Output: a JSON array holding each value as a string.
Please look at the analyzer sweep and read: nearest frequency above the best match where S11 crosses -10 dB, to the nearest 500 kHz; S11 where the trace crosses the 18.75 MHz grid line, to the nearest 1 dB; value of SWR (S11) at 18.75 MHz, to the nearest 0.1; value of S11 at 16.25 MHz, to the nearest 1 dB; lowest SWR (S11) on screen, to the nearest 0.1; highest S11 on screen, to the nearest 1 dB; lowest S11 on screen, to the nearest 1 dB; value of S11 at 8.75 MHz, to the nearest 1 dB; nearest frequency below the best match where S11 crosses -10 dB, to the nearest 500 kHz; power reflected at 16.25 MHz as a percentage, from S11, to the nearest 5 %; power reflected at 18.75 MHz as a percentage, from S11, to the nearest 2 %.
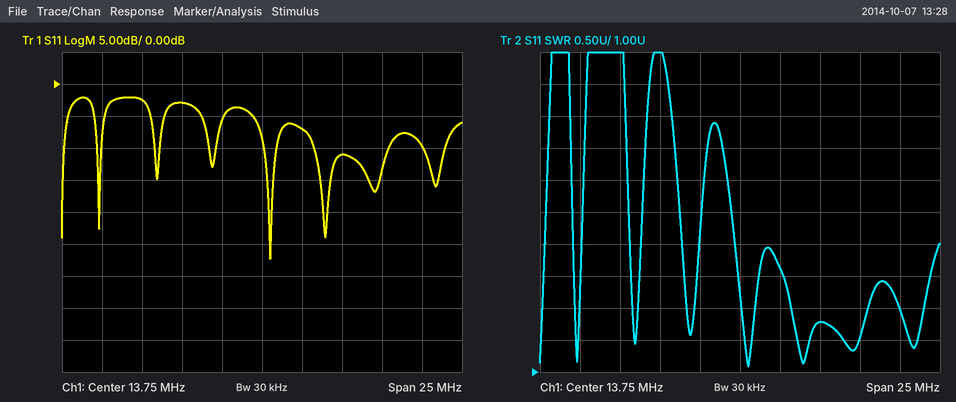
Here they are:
["14.5 MHz", "-11 dB", "1.8", "-7 dB", "1.1", "-2 dB", "-27 dB", "-3 dB", "14.0 MHz", "20 %", "8 %"]
